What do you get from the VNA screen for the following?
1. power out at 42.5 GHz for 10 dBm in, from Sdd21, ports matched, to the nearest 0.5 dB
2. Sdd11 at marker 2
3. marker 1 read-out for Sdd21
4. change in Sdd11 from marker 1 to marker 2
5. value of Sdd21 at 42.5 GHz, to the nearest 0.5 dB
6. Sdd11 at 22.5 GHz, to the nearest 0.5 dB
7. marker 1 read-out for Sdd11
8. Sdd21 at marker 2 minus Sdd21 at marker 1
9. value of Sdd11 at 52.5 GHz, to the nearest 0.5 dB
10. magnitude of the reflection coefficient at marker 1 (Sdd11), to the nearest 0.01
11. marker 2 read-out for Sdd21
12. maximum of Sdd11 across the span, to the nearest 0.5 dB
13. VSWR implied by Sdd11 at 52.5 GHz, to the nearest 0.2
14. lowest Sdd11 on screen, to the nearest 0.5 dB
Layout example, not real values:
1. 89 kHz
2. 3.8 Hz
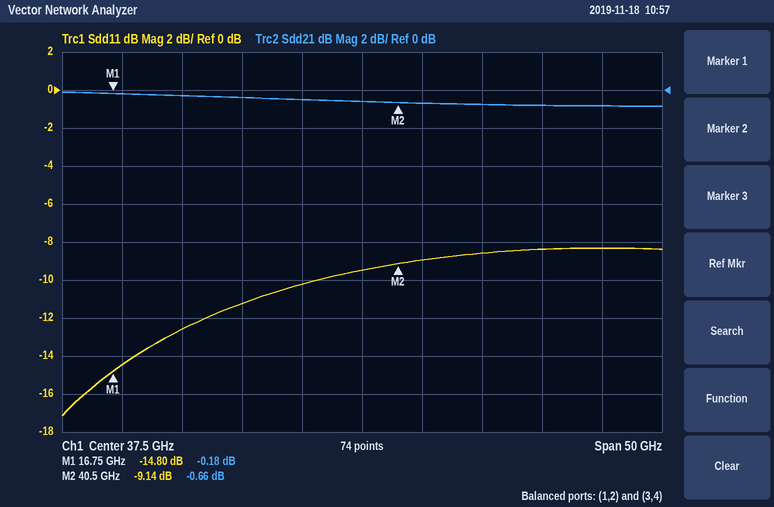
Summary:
1. 9.5 dBm
2. -9.14 dB
3. -0.18 dB
4. 5.66 dB
5. -0.5 dB
6. -12.5 dB
7. -14.80 dB
8. -0.48 dB
9. -8.5 dB
10. 0.18
11. -0.66 dB
12. -8.5 dB
13. 2.2
14. -17.0 dB
